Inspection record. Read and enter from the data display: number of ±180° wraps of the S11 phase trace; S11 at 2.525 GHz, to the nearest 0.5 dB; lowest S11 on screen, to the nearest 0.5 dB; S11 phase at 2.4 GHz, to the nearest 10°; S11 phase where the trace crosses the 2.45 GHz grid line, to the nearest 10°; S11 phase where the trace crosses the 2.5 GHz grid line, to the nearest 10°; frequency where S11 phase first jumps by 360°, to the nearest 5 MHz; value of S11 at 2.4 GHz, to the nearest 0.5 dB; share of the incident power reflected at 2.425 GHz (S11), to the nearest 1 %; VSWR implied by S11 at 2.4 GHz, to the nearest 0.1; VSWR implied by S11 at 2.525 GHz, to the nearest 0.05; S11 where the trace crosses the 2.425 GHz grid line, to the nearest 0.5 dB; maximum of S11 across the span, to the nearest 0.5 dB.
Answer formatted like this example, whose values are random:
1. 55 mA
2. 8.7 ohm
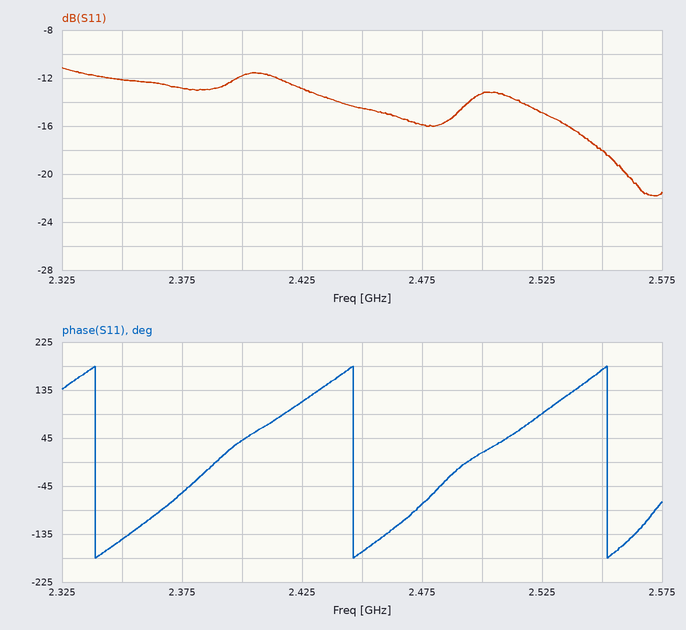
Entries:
1. 3
2. -15.0 dB
3. -22.0 dB
4. 40°
5. -170°
6. 20°
7. 2.340 GHz
8. -12.0 dB
9. 5 %
10. 1.7
11. 1.45
12. -13.0 dB
13. -11.0 dB
